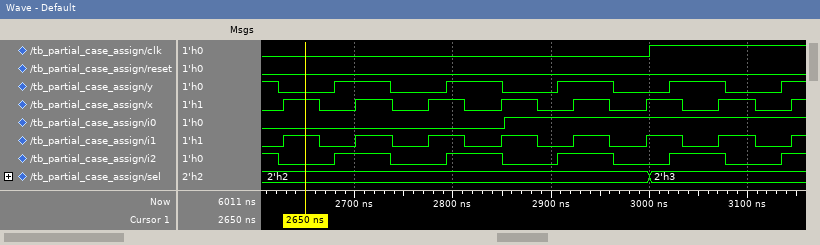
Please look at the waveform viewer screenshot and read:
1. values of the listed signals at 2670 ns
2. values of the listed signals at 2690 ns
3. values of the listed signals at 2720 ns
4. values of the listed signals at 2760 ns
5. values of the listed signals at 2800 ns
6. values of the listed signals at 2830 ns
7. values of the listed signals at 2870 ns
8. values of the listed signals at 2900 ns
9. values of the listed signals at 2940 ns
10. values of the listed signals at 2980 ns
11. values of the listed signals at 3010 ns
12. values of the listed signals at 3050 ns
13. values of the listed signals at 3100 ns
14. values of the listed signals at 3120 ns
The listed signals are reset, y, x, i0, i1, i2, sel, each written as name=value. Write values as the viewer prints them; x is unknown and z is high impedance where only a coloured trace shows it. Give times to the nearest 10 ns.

reset=0, y=0, x=0, i0=0, i1=0, i2=0, sel=2'h2
reset=0, y=1, x=0, i0=0, i1=0, i2=1, sel=2'h2
reset=0, y=1, x=1, i0=0, i1=1, i2=1, sel=2'h2
reset=0, y=0, x=0, i0=0, i1=0, i2=0, sel=2'h2
reset=0, y=1, x=1, i0=0, i1=1, i2=1, sel=2'h2
reset=0, y=1, x=0, i0=0, i1=0, i2=1, sel=2'h2
reset=0, y=0, x=1, i0=1, i1=1, i2=0, sel=2'h2
reset=0, y=0, x=0, i0=1, i1=0, i2=0, sel=2'h2
reset=0, y=1, x=1, i0=1, i1=1, i2=1, sel=2'h2
reset=0, y=0, x=0, i0=1, i1=0, i2=0, sel=2'h2
reset=0, y=0, x=1, i0=1, i1=1, i2=0, sel=2'h3
reset=0, y=1, x=0, i0=1, i1=0, i2=1, sel=2'h3
reset=0, y=0, x=1, i0=1, i1=1, i2=0, sel=2'h3
reset=0, y=0, x=0, i0=1, i1=0, i2=0, sel=2'h3
